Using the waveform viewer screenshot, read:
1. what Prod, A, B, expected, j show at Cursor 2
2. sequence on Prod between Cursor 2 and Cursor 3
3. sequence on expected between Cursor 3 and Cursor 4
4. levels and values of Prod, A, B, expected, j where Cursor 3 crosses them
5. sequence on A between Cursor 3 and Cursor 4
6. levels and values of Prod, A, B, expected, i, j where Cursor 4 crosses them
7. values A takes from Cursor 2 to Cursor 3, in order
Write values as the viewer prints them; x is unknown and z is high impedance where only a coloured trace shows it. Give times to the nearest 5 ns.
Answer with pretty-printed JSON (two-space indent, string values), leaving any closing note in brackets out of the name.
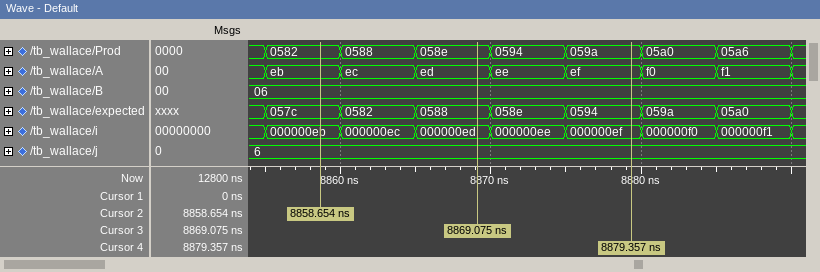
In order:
{
  "what Prod, A, B, expected, j show at Cursor 2": "Prod=0582, A=eb, B=06, expected=057c, j=6",
  "sequence on Prod between Cursor 2 and Cursor 3": "0582, 0588, 058e",
  "sequence on expected between Cursor 3 and Cursor 4": "0588, 058e, 0594",
  "levels and values of Prod, A, B, expected, j where Cursor 3 crosses them": "Prod=058e, A=ed, B=06, expected=0588, j=6",
  "sequence on A between Cursor 3 and Cursor 4": "ed, ee, ef",
  "levels and values of Prod, A, B, expected, i, j where Cursor 4 crosses them": "Prod=059a, A=ef, B=06, expected=0594, i=000000ef, j=6",
  "values A takes from Cursor 2 to Cursor 3, in order": "eb, ec, ed"
}
